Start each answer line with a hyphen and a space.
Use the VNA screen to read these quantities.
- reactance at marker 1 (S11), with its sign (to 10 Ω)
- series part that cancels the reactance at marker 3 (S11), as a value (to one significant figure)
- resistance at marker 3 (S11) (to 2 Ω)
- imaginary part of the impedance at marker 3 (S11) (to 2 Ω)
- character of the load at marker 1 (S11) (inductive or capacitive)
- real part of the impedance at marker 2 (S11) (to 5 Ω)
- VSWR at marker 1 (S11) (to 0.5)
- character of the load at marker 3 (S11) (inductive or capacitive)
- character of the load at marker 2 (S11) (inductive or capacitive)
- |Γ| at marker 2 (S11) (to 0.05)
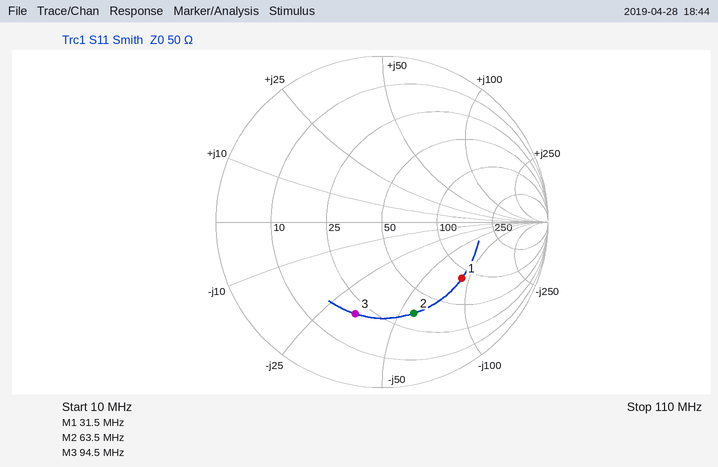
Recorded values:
- -90 Ω
- 60 nH
- 20 Ω
- -34 Ω
- capacitive
- 35 Ω
- 4.0
- capacitive
- capacitive
- 0.60
